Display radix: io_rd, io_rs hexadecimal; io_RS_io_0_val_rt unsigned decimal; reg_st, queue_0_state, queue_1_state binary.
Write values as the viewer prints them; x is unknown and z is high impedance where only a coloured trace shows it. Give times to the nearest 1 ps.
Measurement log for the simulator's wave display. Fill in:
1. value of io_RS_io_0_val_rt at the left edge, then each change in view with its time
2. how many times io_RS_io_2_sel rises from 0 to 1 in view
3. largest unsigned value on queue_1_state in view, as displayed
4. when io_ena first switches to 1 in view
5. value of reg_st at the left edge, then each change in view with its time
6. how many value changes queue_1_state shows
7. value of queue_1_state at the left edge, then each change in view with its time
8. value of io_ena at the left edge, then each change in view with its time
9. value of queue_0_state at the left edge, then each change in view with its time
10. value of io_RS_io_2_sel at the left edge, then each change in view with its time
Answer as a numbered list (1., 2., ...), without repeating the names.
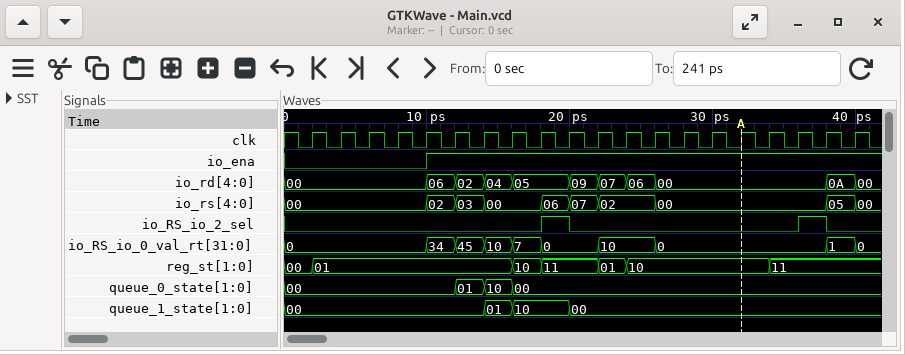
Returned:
1. 0, 34 at 10 ps, 45 at 12 ps, 10 at 14 ps, 7 at 16 ps, 0 at 18 ps, 10 at 22 ps, 0 at 26 ps, 1 at 38 ps, 0 at 40 ps
2. 2
3. 10
4. 10 ps
5. 00, 01 at 2 ps, 10 at 16 ps, 11 at 18 ps, 01 at 22 ps, 10 at 24 ps, 11 at 34 ps
6. 3
7. 00, 01 at 14 ps, 10 at 16 ps, 00 at 20 ps
8. 0, 1 at 10 ps
9. 00, 01 at 12 ps, 10 at 14 ps, 00 at 16 ps
10. 0, 1 at 18 ps, 0 at 20 ps, 1 at 36 ps, 0 at 38 ps
